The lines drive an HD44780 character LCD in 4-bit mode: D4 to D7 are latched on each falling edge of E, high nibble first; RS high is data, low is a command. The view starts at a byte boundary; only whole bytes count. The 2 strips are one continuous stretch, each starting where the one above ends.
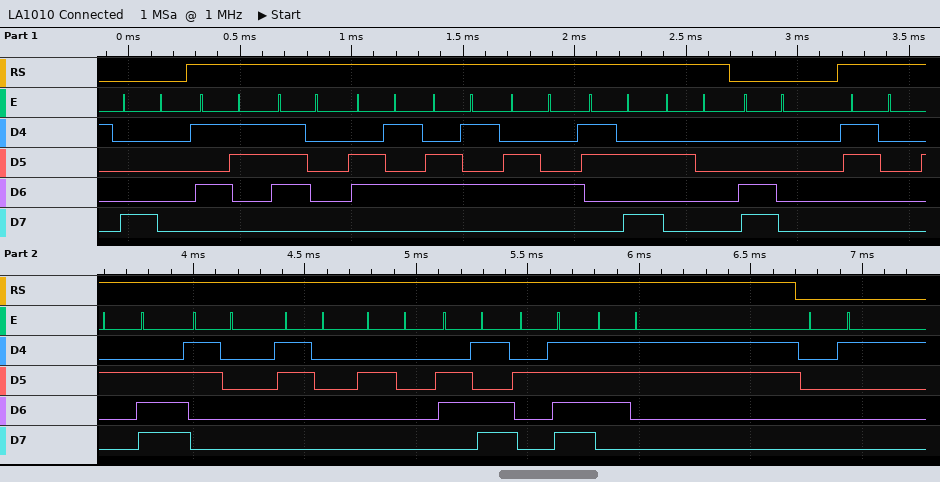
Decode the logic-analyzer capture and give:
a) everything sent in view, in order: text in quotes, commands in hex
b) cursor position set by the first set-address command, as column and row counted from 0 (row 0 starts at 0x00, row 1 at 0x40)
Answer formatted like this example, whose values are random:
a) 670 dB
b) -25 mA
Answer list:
a) 0x80 "Speed: " 0xC0 "0.00 m/s" 0x01
b) column 0, row 0
